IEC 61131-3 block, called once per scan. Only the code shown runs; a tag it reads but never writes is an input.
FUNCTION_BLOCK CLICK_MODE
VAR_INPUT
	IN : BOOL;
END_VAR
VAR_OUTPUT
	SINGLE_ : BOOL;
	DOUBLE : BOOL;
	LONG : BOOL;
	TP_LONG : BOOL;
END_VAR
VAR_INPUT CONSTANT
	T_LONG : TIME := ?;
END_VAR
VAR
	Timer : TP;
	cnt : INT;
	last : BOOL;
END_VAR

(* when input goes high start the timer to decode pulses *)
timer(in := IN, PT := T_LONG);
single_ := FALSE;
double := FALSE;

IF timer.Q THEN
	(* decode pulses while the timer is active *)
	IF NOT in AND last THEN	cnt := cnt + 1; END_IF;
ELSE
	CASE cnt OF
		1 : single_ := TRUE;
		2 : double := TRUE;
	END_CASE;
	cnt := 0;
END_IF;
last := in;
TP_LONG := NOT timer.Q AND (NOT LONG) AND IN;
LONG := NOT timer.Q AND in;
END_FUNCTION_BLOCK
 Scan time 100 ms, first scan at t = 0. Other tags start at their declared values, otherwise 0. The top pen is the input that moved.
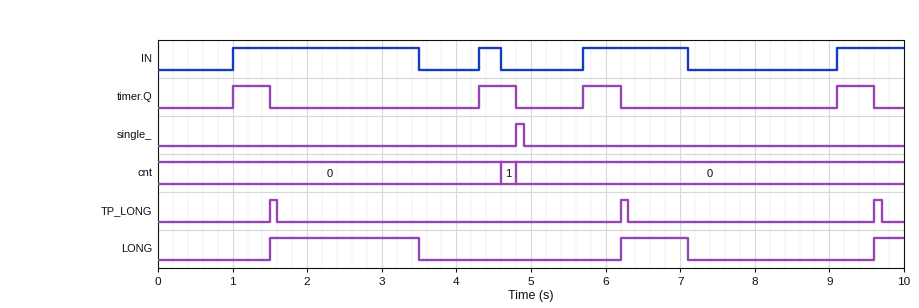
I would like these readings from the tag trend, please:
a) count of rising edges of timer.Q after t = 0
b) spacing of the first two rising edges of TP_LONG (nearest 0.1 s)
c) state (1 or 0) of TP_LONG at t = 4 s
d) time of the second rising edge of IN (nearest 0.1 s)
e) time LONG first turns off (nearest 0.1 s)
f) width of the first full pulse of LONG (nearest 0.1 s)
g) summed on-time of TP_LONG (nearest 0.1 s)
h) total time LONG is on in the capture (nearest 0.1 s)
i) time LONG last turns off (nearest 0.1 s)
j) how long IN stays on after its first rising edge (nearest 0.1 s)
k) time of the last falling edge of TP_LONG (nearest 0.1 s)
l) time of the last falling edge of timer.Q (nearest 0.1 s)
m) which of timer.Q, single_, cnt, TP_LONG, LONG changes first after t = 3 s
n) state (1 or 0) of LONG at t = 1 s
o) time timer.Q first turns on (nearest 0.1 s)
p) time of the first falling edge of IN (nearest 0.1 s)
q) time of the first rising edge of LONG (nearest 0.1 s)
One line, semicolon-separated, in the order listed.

4; 4.7 s; 0; 4.3 s; 3.5 s; 2.0 s; 0.3 s; 3.3 s; 7.1 s; 2.5 s; 9.7 s; 9.6 s; LONG; 0; 1.0 s; 3.5 s; 1.5 s
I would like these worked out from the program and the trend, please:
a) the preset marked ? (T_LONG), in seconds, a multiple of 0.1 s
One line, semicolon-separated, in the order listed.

0.5 s
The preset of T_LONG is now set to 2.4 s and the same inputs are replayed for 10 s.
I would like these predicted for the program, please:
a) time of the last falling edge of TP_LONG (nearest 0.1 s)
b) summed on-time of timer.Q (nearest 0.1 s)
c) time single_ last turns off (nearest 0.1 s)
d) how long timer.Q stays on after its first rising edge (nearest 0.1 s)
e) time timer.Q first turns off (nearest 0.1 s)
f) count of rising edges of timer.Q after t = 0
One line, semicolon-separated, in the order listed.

6.8 s; 5.7 s; 6.8 s; 2.4 s; 3.4 s; 3
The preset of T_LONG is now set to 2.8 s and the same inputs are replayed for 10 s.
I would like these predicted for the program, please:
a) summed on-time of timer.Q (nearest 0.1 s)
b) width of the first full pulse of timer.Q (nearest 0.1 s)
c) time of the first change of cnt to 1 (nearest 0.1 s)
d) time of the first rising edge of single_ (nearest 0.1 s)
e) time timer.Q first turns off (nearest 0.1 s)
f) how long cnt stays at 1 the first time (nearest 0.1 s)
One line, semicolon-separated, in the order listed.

6.5 s; 2.8 s; 3.5 s; 3.8 s; 3.8 s; 0.3 s
